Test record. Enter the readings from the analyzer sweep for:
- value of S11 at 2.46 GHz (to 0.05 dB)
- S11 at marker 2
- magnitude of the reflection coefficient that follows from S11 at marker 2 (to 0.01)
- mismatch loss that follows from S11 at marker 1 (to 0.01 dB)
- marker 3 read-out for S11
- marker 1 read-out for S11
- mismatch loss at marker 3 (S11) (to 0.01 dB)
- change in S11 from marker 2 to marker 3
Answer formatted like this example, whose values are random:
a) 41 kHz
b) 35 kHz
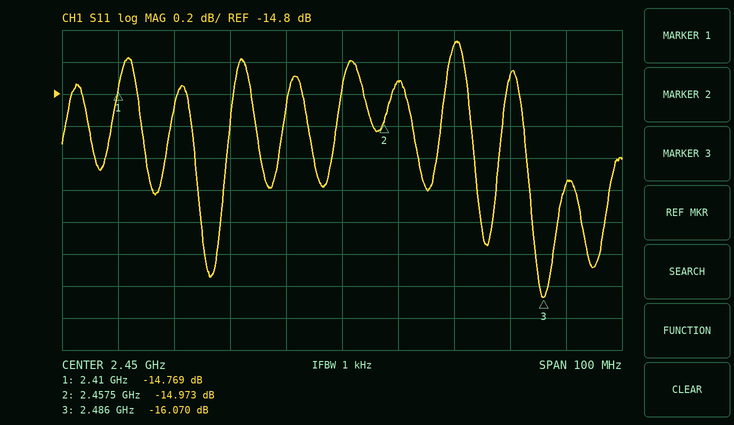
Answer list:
a) -14.70 dB
b) -14.973 dB
c) 0.18
d) 0.15 dB
e) -16.070 dB
f) -14.769 dB
g) 0.11 dB
h) -1.097 dB
